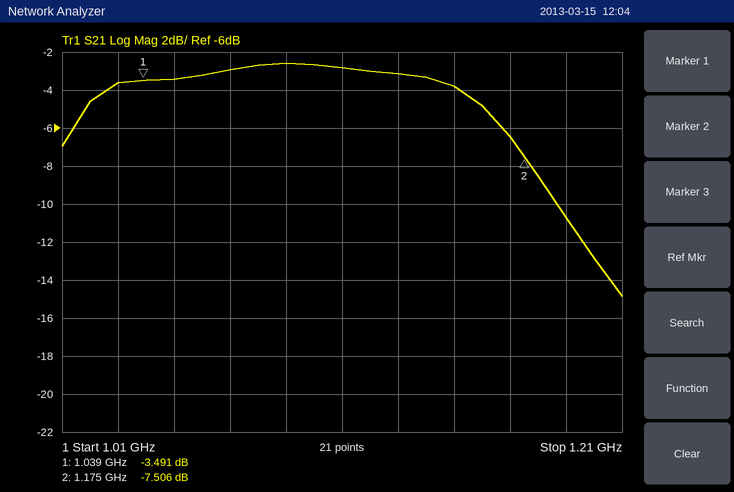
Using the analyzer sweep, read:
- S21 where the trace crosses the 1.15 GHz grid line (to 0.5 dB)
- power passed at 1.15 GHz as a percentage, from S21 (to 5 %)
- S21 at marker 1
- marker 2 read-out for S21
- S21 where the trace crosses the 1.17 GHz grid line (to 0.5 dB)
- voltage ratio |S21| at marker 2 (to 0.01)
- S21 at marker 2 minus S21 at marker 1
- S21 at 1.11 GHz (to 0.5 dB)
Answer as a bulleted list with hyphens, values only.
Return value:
- -4.0 dB
- 40 %
- -3.491 dB
- -7.506 dB
- -6.5 dB
- 0.42
- -4.015 dB
- -3.0 dB
